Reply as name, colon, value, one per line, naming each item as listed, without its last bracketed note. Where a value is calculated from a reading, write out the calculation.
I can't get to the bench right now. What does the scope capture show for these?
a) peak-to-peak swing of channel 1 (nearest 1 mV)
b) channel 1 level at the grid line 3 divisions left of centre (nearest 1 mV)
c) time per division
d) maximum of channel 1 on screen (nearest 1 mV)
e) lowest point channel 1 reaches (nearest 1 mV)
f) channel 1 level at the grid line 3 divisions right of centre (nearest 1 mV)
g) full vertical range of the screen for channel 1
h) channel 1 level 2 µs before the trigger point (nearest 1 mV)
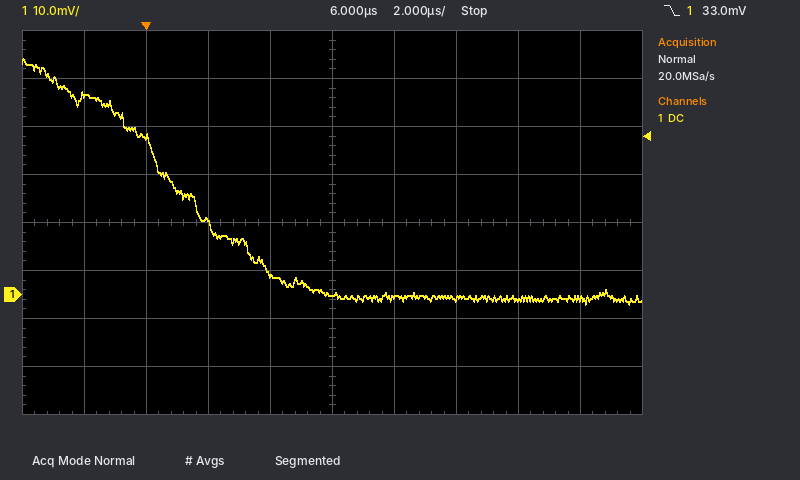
peak-to-peak swing of channel 1: 49 mV − (-2 mV) = 51 mV
channel 1 level at the grid line 3 divisions left of centre: 33 mV
time per division: 2 µs
maximum of channel 1 on screen: 49 mV
lowest point channel 1 reaches: -2 mV
channel 1 level at the grid line 3 divisions right of centre: -1 mV
full vertical range of the screen for channel 1: 80 mV
channel 1 level 2 µs before the trigger point: 42 mV
